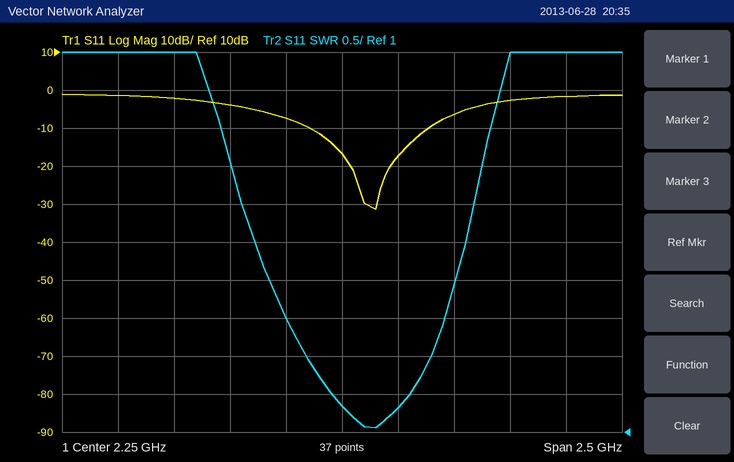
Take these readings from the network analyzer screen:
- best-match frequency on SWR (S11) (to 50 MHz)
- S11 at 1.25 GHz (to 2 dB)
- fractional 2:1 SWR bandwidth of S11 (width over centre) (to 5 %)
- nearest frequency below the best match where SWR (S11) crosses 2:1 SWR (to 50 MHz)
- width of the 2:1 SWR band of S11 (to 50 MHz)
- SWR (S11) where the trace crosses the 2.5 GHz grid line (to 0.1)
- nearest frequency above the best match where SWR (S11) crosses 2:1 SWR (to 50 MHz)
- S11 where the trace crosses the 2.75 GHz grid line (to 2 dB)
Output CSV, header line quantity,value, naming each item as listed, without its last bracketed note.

quantity,value
best-match frequency on SWR (S11),2.40 GHz
S11 at 1.25 GHz,-2 dB
fractional 2:1 SWR bandwidth of S11 (width over centre),25 %
nearest frequency below the best match where SWR (S11) crosses 2:1 SWR,2.10 GHz
width of the 2:1 SWR band of S11,550 MHz
SWR (S11) where the trace crosses the 2.5 GHz grid line,1.3
nearest frequency above the best match where SWR (S11) crosses 2:1 SWR,2.65 GHz
S11 where the trace crosses the 2.75 GHz grid line,-6 dB
